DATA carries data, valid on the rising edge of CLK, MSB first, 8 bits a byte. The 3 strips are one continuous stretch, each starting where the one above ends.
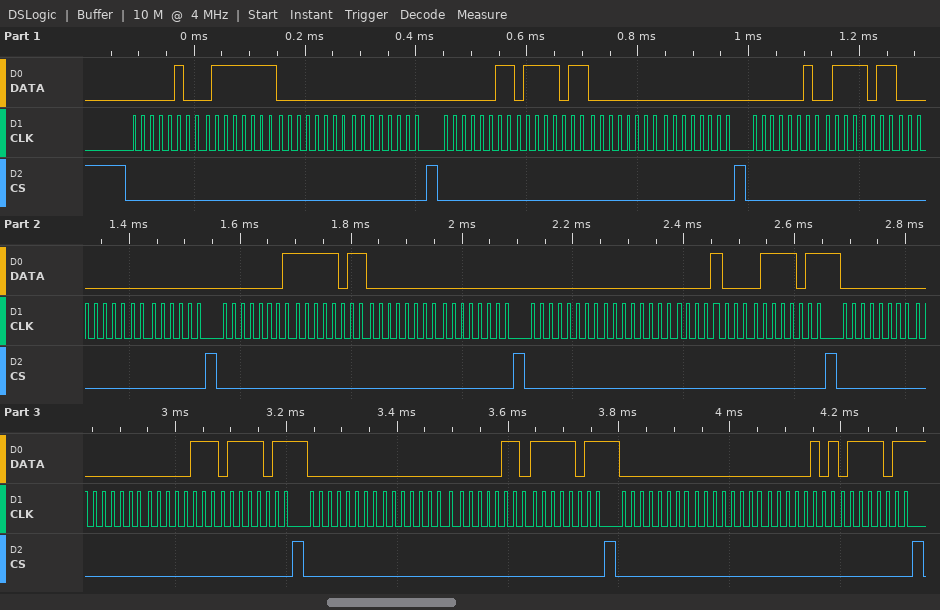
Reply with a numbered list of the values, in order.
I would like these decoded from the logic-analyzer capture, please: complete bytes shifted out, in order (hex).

1. 04 7F 00 00 03 7B 00 00 02 7B 00 00 01 FB 00 00 00 00 08 7B 00 00 07 7B 00 00 06 FB 00 00 05 7B
